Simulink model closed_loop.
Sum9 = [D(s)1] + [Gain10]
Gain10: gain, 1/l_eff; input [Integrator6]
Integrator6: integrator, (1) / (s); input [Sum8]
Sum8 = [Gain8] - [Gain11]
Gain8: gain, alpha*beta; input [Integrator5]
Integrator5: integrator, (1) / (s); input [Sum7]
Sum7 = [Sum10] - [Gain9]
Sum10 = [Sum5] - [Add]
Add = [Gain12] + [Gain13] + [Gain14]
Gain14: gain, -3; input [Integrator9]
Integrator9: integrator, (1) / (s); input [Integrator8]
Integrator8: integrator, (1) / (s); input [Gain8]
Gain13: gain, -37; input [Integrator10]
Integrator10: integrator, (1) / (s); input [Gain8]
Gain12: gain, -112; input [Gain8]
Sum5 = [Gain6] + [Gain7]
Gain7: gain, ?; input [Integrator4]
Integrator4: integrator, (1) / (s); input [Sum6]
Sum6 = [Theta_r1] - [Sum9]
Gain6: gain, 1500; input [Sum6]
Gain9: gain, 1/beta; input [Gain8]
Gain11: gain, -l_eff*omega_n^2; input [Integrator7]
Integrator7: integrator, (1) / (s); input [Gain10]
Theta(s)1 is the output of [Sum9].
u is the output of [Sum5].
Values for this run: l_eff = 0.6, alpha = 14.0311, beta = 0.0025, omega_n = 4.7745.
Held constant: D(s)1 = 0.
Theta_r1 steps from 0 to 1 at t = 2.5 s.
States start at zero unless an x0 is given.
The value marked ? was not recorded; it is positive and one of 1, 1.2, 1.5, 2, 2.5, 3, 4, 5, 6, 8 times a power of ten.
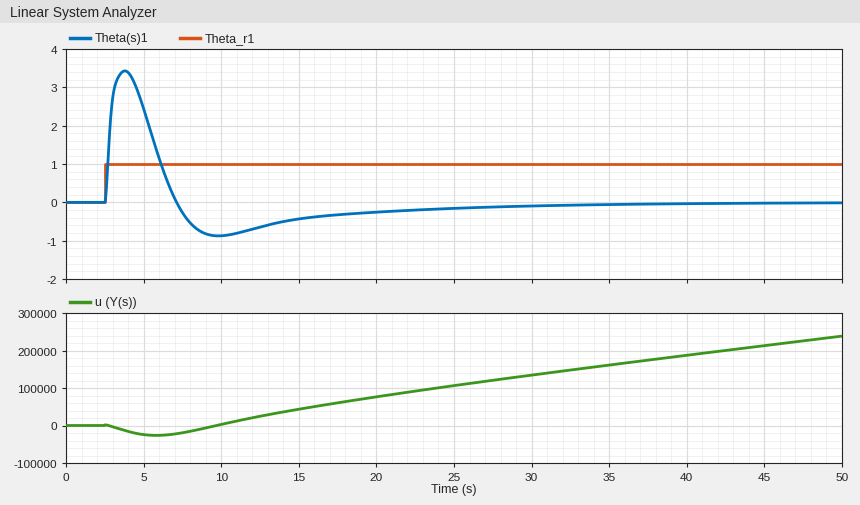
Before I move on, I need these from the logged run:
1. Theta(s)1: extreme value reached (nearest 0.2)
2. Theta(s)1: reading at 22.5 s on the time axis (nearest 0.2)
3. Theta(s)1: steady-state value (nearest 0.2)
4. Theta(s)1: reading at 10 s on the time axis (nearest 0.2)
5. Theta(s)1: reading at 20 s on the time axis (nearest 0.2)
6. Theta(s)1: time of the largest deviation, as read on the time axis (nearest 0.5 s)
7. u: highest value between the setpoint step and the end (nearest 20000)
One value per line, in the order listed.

3.4
-0.2
0.0
-0.8
-0.2
4.0 s
240000
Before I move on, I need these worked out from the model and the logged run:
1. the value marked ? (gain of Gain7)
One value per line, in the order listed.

5000
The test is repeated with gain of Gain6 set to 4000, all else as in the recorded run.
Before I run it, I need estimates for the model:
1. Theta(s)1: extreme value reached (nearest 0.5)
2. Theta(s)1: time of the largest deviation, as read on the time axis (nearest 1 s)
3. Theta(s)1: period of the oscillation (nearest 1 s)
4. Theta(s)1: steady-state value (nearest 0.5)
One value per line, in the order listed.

2.5
5 s
19 s
0.0
